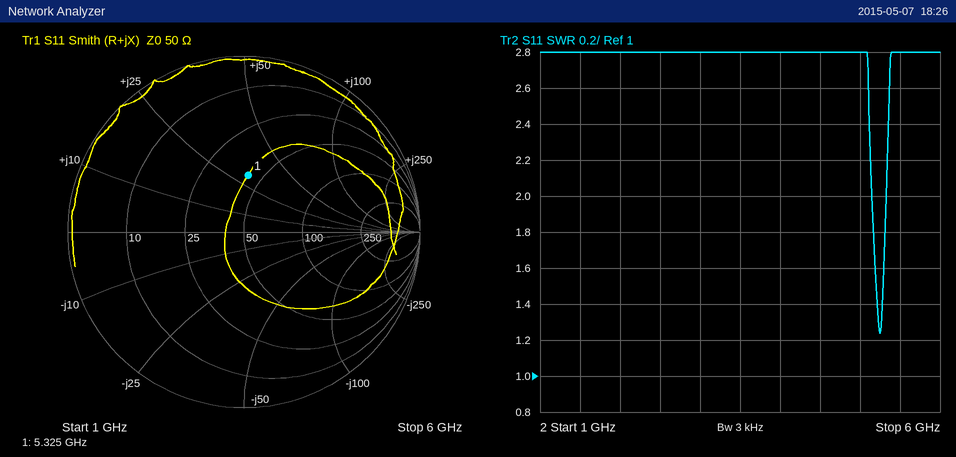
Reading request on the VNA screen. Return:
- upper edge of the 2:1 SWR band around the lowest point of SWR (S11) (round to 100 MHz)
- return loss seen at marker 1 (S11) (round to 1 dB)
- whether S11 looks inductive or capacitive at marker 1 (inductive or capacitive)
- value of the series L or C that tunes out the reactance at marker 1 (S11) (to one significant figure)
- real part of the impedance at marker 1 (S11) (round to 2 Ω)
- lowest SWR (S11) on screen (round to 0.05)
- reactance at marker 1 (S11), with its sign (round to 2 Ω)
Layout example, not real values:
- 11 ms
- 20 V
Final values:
- 5.3 GHz
- 10 dB
- inductive
- 1.0 pF
- 42 Ω
- 1.25
- +30 Ω
